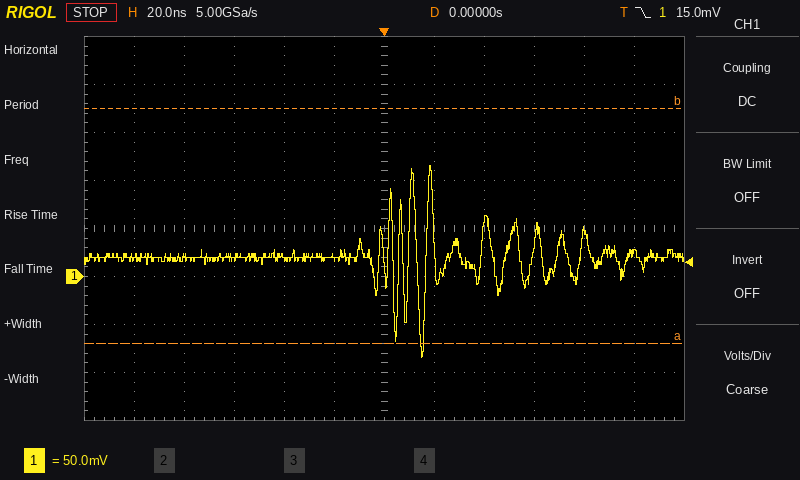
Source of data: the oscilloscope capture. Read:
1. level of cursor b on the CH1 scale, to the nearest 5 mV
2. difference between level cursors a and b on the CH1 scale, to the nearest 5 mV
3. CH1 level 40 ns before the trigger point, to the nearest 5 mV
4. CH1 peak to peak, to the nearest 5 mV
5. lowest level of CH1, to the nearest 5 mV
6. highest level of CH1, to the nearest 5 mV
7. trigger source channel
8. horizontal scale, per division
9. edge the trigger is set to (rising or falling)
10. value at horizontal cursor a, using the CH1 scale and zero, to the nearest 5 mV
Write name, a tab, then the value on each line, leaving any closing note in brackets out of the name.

level of cursor b on the CH1 scale, to the nearest 5 mV	175 mV
difference between level cursors a and b on the CH1 scale, to the nearest 5 mV	245 mV
CH1 level 40 ns before the trigger point, to the nearest 5 mV	20 mV
CH1 peak to peak, to the nearest 5 mV	200 mV
lowest level of CH1, to the nearest 5 mV	-85 mV
highest level of CH1, to the nearest 5 mV	115 mV
trigger source channel	CH1
horizontal scale, per division	20 ns
edge the trigger is set to	falling
value at horizontal cursor a, using the CH1 scale and zero, to the nearest 5 mV	-70 mV
